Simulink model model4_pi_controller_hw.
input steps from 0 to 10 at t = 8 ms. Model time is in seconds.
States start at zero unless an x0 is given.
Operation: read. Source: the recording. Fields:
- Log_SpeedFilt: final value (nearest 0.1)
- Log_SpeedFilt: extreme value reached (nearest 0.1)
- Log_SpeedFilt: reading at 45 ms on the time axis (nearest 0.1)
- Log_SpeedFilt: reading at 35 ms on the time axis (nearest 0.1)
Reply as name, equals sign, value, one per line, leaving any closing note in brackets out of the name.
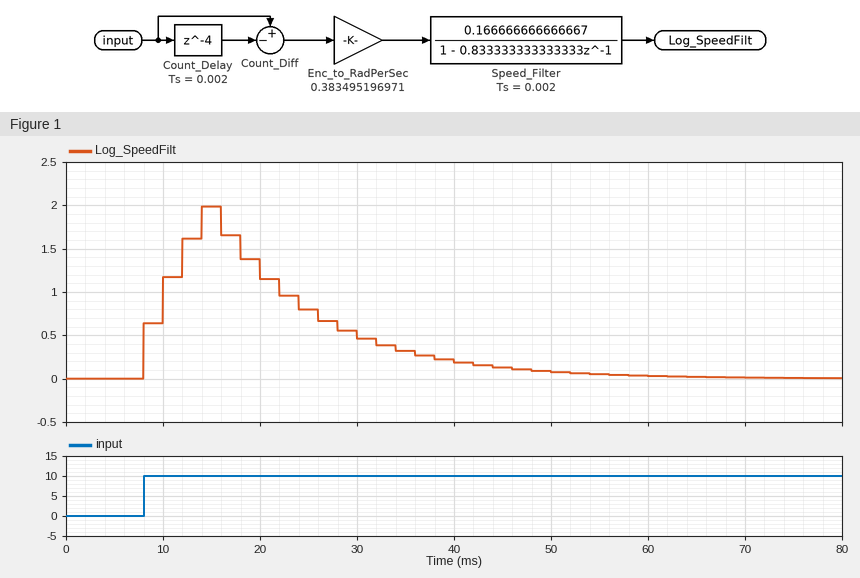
Log_SpeedFilt: final value = 0.0
Log_SpeedFilt: extreme value reached = 2.0
Log_SpeedFilt: reading at 45 ms on the time axis = 0.1
Log_SpeedFilt: reading at 35 ms on the time axis = 0.3
